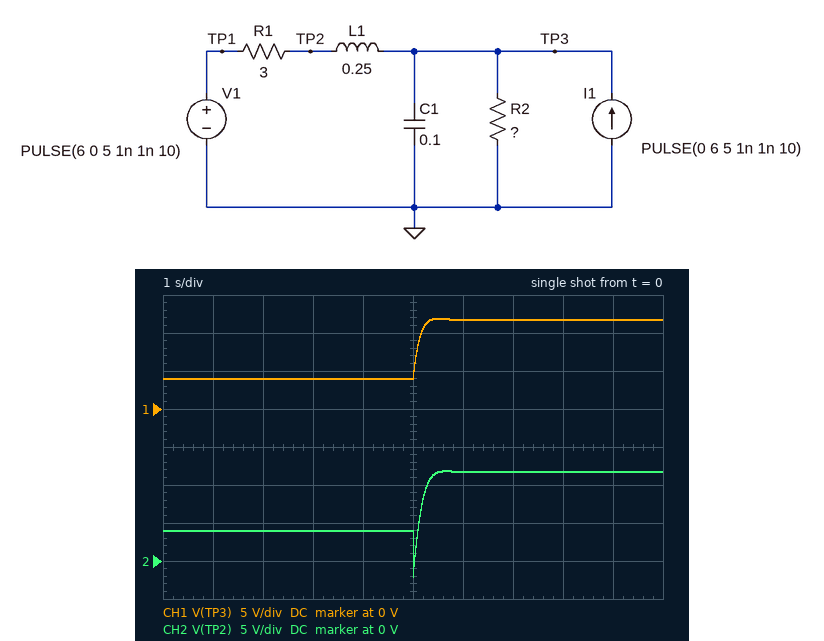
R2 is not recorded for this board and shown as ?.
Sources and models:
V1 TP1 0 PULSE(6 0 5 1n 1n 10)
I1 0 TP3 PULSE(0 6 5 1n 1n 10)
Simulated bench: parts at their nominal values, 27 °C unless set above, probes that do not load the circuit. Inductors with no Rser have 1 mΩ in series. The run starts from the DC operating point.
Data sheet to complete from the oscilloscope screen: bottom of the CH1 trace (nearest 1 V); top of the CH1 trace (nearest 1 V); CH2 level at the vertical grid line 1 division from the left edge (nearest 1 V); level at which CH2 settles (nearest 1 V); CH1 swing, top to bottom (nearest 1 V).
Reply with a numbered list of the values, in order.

1. 4 V
2. 12 V
3. 4 V
4. 12 V
5. 8 V
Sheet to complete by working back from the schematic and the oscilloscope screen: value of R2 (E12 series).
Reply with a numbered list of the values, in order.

1. 5.6 Ω
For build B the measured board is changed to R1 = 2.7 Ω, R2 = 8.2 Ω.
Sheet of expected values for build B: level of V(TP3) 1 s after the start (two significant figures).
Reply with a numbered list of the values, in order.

1. 4.5 V
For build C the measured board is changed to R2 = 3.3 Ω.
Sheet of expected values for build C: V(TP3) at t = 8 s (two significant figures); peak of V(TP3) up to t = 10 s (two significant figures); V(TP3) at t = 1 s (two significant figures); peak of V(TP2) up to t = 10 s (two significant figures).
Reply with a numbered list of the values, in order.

1. 9.4 V
2. 9.6 V
3. 3.1 V
4. 9.5 V
